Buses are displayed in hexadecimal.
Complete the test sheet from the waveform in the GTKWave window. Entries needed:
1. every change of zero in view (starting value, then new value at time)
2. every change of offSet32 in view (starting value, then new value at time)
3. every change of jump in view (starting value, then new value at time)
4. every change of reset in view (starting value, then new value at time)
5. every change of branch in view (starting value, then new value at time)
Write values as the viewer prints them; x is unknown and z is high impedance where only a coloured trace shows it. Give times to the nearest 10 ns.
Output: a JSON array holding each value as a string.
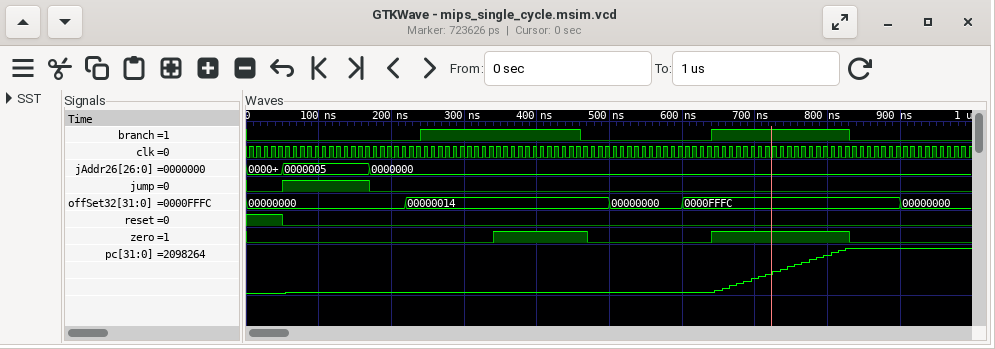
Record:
["0, 1 at 340 ns, 0 at 470 ns, 1 at 640 ns, 0 at 830 ns", "00000000, 00000014 at 220 ns, 00000000 at 500 ns, 0000FFFC at 600 ns, 00000000 at 900 ns", "0, 1 at 50 ns, 0 at 170 ns", "1, 0 at 50 ns", "0, 1 at 240 ns, 0 at 460 ns, 1 at 640 ns, 0 at 830 ns"]
